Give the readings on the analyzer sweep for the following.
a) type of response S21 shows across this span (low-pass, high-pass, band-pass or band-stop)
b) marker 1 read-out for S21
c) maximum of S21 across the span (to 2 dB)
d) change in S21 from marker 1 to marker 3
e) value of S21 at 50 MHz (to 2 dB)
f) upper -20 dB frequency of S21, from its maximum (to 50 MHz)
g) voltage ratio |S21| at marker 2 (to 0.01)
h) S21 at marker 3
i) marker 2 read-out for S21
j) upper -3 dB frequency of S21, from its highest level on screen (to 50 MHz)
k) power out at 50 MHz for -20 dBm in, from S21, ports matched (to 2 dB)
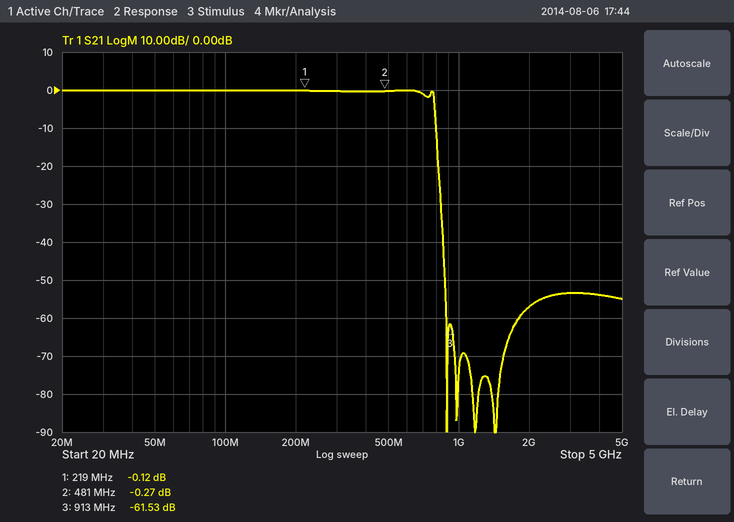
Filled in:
low-pass
-0.12 dB
0 dB
-61.41 dB
0 dB
800 MHz
0.97
-61.53 dB
-0.27 dB
800 MHz
-20 dBm
